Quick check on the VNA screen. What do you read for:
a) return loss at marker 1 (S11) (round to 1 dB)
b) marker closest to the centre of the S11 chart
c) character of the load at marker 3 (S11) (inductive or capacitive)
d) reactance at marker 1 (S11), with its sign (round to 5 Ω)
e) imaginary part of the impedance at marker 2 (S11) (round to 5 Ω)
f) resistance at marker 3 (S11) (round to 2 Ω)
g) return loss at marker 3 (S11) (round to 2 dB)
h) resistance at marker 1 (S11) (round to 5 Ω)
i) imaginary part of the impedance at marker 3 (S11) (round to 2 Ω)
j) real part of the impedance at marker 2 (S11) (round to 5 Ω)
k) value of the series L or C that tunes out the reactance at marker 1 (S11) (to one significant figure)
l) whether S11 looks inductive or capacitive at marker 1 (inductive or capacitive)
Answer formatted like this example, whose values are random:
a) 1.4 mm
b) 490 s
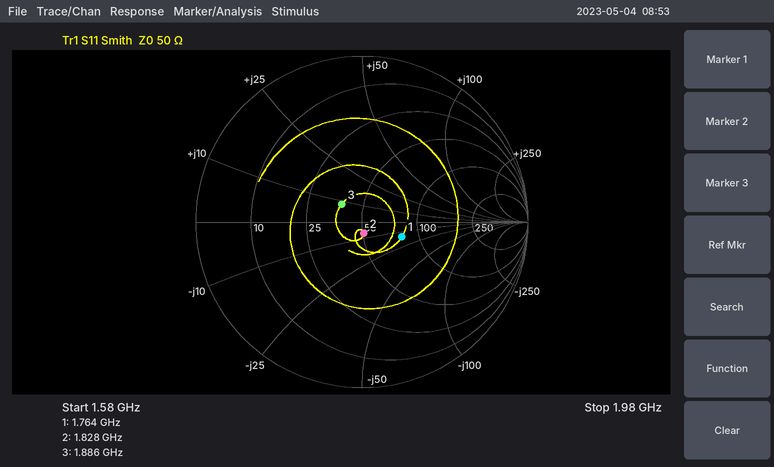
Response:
a) 12 dB
b) marker 2
c) inductive
d) -15 Ω
e) -5 Ω
f) 38 Ω
g) 16 dB
h) 80 Ω
i) +8 Ω
j) 50 Ω
k) 1 nH
l) capacitive
